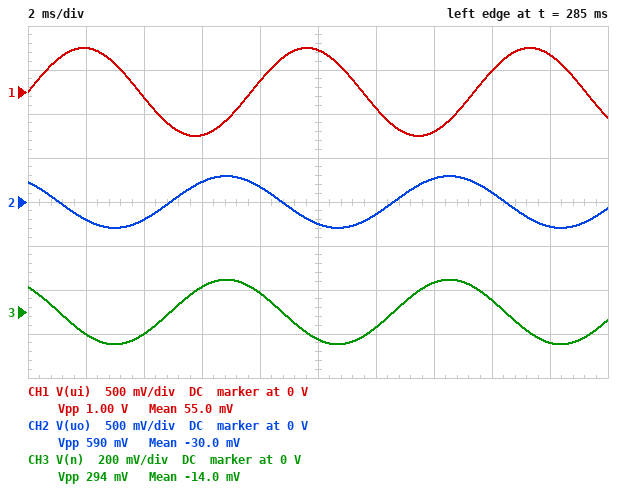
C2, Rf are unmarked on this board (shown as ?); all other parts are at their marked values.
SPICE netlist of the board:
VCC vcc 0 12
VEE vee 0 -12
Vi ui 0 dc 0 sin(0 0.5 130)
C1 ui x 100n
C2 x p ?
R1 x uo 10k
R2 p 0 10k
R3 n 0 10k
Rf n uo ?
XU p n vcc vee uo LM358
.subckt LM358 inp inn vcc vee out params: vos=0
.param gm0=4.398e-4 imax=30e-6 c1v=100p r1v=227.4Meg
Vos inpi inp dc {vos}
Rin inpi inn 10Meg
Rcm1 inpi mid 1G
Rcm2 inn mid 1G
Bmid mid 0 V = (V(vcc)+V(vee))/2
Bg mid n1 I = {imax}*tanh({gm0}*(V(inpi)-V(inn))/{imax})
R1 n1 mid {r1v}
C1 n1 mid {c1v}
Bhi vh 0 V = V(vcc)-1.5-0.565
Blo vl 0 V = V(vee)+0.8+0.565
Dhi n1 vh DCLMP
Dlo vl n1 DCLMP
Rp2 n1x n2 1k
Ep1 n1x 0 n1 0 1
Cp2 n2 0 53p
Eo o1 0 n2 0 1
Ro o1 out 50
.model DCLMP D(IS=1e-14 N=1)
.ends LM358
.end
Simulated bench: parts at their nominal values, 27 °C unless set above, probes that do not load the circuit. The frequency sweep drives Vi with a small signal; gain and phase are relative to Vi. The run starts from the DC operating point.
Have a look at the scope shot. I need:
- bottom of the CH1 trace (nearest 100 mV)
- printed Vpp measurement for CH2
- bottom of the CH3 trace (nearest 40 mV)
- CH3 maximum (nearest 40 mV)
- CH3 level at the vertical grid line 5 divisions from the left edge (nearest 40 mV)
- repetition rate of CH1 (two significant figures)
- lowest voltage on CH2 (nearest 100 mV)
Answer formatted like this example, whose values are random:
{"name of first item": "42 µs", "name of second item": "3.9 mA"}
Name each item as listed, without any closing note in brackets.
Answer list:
{"bottom of the CH1 trace": "-500 mV", "printed Vpp measurement for CH2": "590 mV", "bottom of the CH3 trace": "-160 mV", "CH3 maximum": "160 mV", "CH3 level at the vertical grid line 5 divisions from the left edge": "-120 mV", "repetition rate of CH1": "130 Hz", "lowest voltage on CH2": "-300 mV"}
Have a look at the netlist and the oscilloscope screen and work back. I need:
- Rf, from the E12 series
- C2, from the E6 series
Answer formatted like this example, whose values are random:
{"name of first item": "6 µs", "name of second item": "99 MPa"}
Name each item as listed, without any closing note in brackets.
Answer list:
{"Rf, from the E12 series": "10 kΩ", "C2, from the E6 series": "47 nF"}
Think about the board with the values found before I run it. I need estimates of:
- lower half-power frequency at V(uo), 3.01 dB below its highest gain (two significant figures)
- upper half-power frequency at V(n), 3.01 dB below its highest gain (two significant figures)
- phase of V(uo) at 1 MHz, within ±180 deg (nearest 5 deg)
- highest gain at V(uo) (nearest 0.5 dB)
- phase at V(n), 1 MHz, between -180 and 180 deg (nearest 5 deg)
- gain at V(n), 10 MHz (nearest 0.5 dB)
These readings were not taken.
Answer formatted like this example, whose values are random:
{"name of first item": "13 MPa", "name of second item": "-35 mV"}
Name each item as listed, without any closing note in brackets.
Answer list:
{"lower half-power frequency at V(uo), 3.01 dB below its highest gain": "240 Hz", "upper half-power frequency at V(n), 3.01 dB below its highest gain": "390 kHz", "phase of V(uo) at 1 MHz, within ±180 deg": "-90 deg", "highest gain at V(uo)": "6.0 dB", "phase at V(n), 1 MHz, between -180 and 180 deg": "-90 deg", "gain at V(n), 10 MHz": "-43.0 dB"}
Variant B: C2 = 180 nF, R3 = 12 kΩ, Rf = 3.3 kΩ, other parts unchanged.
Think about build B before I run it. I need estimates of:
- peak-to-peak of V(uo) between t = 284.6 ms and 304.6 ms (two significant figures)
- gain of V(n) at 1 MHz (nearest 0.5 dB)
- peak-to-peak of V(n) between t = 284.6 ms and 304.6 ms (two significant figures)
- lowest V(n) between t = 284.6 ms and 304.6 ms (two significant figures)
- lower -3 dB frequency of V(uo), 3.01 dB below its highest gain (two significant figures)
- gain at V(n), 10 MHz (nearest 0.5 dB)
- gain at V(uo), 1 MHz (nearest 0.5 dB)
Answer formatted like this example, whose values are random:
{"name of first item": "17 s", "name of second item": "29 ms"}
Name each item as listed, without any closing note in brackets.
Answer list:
{"peak-to-peak of V(uo) between t = 284.6 ms and 304.6 ms": "810 mV", "gain of V(n) at 1 MHz": "-5.5 dB", "peak-to-peak of V(n) between t = 284.6 ms and 304.6 ms": "630 mV", "lowest V(n) between t = 284.6 ms and 304.6 ms": "-320 mV", "lower -3 dB frequency of V(uo), 3.01 dB below its highest gain": "150 Hz", "gain at V(n), 10 MHz": "-38.5 dB", "gain at V(uo), 1 MHz": "-3.5 dB"}
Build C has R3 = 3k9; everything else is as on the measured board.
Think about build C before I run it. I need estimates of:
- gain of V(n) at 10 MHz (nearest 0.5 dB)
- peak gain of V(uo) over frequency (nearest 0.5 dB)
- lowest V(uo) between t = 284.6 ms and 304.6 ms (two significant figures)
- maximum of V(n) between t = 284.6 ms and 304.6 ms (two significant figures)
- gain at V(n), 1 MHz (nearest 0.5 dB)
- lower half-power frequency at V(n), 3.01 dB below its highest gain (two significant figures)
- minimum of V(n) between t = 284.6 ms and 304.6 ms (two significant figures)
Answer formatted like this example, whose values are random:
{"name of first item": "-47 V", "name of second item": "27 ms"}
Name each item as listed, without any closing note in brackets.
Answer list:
{"gain of V(n) at 10 MHz": "-48.0 dB", "peak gain of V(uo) over frequency": "19.5 dB", "lowest V(uo) between t = 284.6 ms and 304.6 ms": "-780 mV", "maximum of V(n) between t = 284.6 ms and 304.6 ms": "220 mV", "gain at V(n), 1 MHz": "-14.5 dB", "lower half-power frequency at V(n), 3.01 dB below its highest gain": "200 Hz", "minimum of V(n) between t = 284.6 ms and 304.6 ms": "-220 mV"}
